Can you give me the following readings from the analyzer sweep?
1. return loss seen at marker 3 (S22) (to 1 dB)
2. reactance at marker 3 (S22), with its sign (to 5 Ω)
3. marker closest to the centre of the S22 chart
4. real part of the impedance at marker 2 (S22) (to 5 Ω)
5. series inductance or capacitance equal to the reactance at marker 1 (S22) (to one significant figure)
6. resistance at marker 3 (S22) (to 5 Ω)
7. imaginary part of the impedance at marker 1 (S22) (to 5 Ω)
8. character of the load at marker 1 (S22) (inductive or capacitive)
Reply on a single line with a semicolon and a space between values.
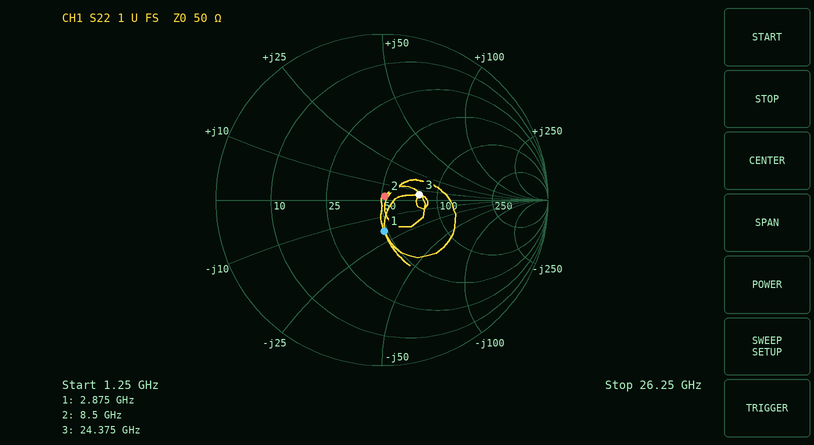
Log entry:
13 dB; +5 Ω; marker 2; 50 Ω; 3 pF; 80 Ω; -20 Ω; capacitive
